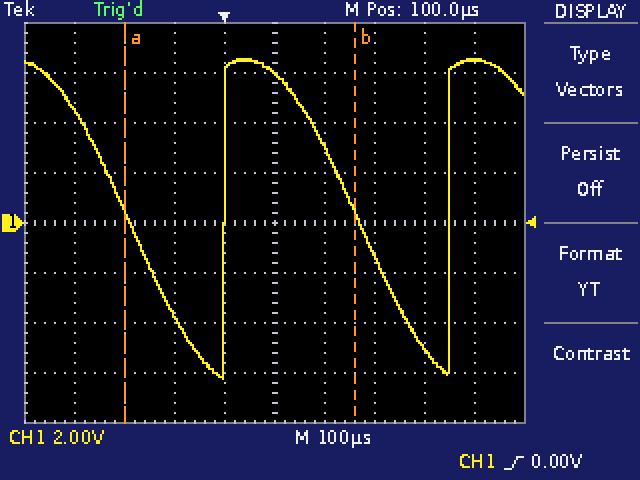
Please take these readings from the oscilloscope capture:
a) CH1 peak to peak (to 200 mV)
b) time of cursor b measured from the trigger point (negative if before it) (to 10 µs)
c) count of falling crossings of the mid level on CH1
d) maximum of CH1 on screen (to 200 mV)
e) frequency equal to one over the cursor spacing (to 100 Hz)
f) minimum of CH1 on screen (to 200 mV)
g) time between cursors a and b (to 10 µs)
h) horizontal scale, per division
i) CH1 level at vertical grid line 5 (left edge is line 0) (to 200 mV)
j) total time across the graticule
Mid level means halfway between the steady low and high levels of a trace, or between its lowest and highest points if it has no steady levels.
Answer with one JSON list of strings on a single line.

["12.8 V", "+260 µs", "2", "6.6 V", "2.2 kHz", "-6.2 V", "460 µs", "100 µs", "6.0 V", "1 ms"]
